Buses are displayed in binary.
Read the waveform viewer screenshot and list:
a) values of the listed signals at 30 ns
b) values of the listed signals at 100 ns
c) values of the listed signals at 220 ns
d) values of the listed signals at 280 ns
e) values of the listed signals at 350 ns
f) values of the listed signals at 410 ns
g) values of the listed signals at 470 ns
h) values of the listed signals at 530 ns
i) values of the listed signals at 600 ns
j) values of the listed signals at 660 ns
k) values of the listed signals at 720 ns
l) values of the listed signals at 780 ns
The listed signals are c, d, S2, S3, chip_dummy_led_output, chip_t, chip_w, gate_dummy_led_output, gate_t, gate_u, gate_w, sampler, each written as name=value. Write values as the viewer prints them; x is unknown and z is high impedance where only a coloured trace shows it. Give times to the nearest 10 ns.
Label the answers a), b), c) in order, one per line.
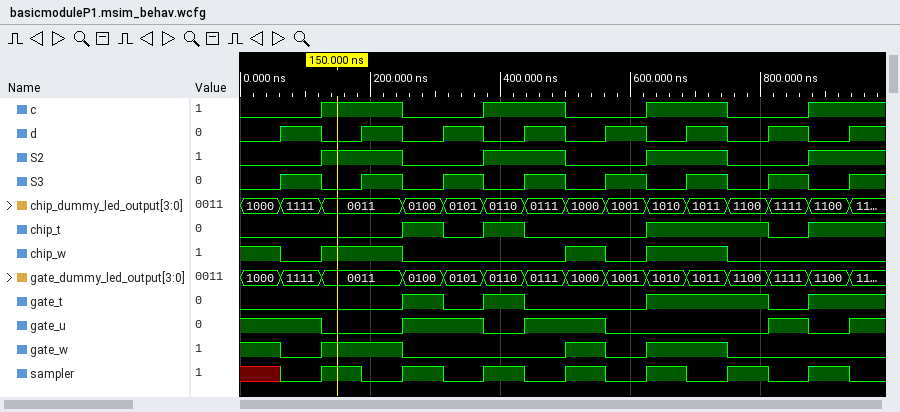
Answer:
a) c=0, d=0, S2=0, S3=0, chip_dummy_led_output=1000, chip_t=0, chip_w=1, gate_dummy_led_output=1000, gate_t=0, gate_u=1, gate_w=1, sampler=x
b) c=0, d=1, S2=0, S3=1, chip_dummy_led_output=1111, chip_t=0, chip_w=0, gate_dummy_led_output=1111, gate_t=0, gate_u=1, gate_w=0, sampler=0
c) c=1, d=1, S2=1, S3=1, chip_dummy_led_output=0011, chip_t=0, chip_w=1, gate_dummy_led_output=0011, gate_t=0, gate_u=0, gate_w=1, sampler=0
d) c=0, d=0, S2=0, S3=0, chip_dummy_led_output=0100, chip_t=1, chip_w=0, gate_dummy_led_output=0100, gate_t=1, gate_u=1, gate_w=0, sampler=1
e) c=0, d=1, S2=0, S3=1, chip_dummy_led_output=0101, chip_t=0, chip_w=0, gate_dummy_led_output=0101, gate_t=0, gate_u=1, gate_w=0, sampler=0
f) c=1, d=0, S2=1, S3=0, chip_dummy_led_output=0110, chip_t=1, chip_w=0, gate_dummy_led_output=0110, gate_t=1, gate_u=0, gate_w=0, sampler=1
g) c=1, d=1, S2=1, S3=1, chip_dummy_led_output=0111, chip_t=0, chip_w=0, gate_dummy_led_output=0111, gate_t=0, gate_u=1, gate_w=0, sampler=0
h) c=0, d=0, S2=0, S3=0, chip_dummy_led_output=1000, chip_t=0, chip_w=1, gate_dummy_led_output=1000, gate_t=0, gate_u=1, gate_w=1, sampler=1
i) c=0, d=1, S2=0, S3=1, chip_dummy_led_output=1001, chip_t=0, chip_w=0, gate_dummy_led_output=1001, gate_t=0, gate_u=0, gate_w=0, sampler=0
j) c=1, d=0, S2=1, S3=0, chip_dummy_led_output=1010, chip_t=1, chip_w=1, gate_dummy_led_output=1010, gate_t=1, gate_u=0, gate_w=1, sampler=1
k) c=1, d=1, S2=1, S3=1, chip_dummy_led_output=1011, chip_t=1, chip_w=1, gate_dummy_led_output=1011, gate_t=1, gate_u=0, gate_w=1, sampler=0
l) c=0, d=0, S2=0, S3=0, chip_dummy_led_output=1100, chip_t=1, chip_w=0, gate_dummy_led_output=1100, gate_t=1, gate_u=0, gate_w=0, sampler=1
